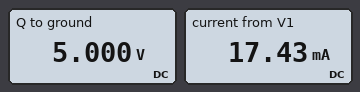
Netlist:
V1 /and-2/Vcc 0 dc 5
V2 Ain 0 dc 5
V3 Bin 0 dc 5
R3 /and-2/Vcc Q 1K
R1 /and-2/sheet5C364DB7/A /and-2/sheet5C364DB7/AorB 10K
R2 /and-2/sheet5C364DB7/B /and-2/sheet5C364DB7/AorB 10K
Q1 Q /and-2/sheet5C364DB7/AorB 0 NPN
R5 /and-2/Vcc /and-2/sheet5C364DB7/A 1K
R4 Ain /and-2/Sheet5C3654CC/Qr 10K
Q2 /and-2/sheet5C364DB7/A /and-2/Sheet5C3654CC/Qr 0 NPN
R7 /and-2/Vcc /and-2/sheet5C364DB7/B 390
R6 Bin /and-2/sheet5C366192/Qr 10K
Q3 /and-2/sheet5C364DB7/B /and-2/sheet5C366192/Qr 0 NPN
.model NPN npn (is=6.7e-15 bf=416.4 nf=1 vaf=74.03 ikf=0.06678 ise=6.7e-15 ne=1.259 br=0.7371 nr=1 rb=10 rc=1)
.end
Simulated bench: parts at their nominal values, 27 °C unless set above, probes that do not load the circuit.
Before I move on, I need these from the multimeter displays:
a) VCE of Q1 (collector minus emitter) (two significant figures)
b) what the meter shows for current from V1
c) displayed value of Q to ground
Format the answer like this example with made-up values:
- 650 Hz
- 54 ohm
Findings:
- 5.0 V
- 17.43 mA
- 5.000 V
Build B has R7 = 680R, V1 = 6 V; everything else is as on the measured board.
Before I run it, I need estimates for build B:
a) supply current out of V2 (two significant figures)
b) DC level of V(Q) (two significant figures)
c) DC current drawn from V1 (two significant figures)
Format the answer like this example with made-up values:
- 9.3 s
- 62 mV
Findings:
- 430 µA
- 6.0 V
- 15 mA
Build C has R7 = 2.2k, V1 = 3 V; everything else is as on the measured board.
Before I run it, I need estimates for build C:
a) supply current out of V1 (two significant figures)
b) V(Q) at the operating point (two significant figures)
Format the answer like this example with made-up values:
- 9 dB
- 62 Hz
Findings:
- 4.3 mA
- 3.0 V
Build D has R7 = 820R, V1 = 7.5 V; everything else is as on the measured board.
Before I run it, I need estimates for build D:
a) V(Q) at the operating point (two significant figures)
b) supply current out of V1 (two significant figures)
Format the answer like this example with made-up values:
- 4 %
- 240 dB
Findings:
- 7.5 V
- 16 mA
